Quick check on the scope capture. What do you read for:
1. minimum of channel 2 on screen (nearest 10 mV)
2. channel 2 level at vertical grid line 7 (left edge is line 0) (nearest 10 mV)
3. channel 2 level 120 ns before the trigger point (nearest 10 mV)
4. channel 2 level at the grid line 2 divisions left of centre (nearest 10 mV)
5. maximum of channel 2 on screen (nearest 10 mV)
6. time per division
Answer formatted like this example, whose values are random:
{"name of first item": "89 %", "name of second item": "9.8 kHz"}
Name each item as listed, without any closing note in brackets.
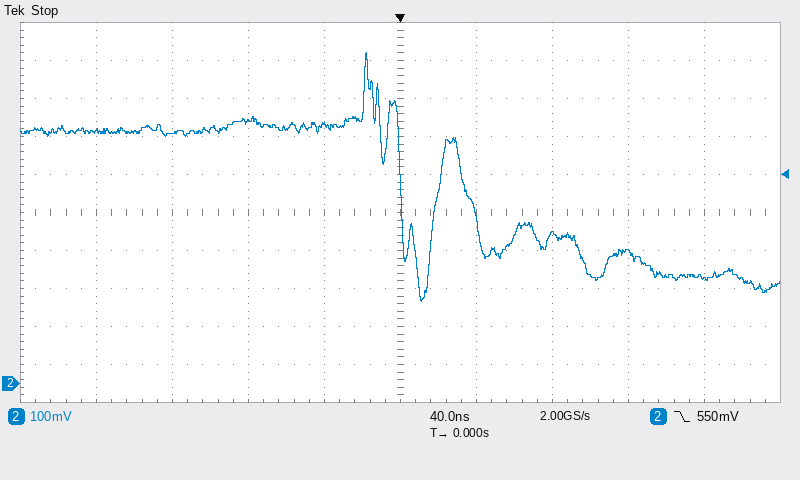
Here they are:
{"minimum of channel 2 on screen": "220 mV", "channel 2 level at vertical grid line 7 (left edge is line 0)": "390 mV", "channel 2 level 120 ns before the trigger point": "660 mV", "channel 2 level at the grid line 2 divisions left of centre": "690 mV", "maximum of channel 2 on screen": "870 mV", "time per division": "40 ns"}
